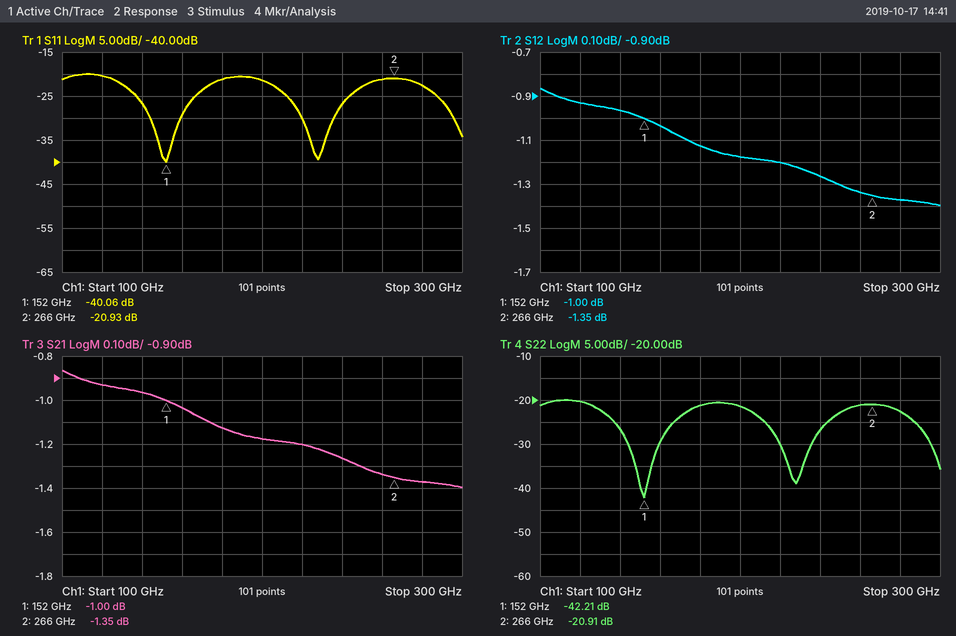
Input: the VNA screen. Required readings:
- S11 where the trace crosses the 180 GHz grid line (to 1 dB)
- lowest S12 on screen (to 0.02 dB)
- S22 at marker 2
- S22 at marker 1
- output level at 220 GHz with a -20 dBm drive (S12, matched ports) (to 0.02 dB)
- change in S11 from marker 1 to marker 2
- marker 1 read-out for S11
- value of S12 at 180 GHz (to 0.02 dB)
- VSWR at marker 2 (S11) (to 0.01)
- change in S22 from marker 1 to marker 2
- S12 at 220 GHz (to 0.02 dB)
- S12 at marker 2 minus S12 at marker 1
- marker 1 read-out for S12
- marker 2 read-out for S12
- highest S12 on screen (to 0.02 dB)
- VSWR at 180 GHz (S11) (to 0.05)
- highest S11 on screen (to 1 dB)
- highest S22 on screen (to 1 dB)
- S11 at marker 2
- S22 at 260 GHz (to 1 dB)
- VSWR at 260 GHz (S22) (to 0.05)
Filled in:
-21 dB
-1.40 dB
-20.91 dB
-42.21 dB
-21.20 dBm
19.13 dB
-40.06 dB
-1.12 dB
1.20
21.30 dB
-1.20 dB
-0.35 dB
-1.00 dB
-1.35 dB
-0.86 dB
1.20
-20 dB
-20 dB
-20.93 dB
-21 dB
1.20
